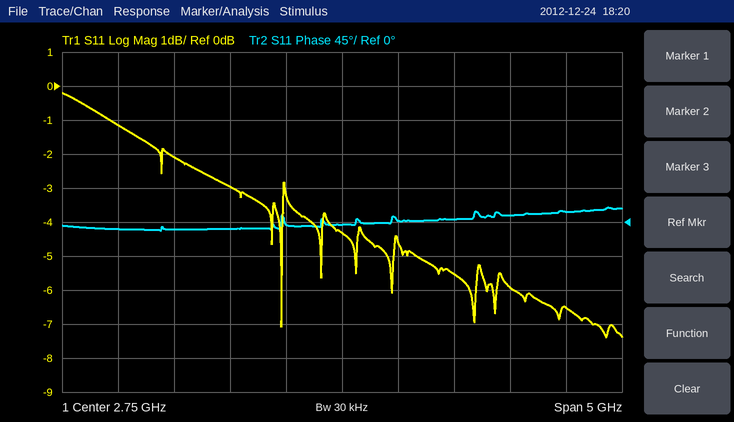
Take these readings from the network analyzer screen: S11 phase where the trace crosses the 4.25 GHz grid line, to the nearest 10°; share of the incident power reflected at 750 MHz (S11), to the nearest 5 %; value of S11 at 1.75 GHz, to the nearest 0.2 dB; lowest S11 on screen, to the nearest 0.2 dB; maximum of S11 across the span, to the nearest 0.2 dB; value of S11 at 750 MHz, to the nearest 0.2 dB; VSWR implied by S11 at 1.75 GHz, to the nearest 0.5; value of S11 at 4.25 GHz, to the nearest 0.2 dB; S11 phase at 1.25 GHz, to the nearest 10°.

10°
75 %
-3.0 dB
-7.4 dB
-0.2 dB
-1.2 dB
6.0
-6.0 dB
-10°
